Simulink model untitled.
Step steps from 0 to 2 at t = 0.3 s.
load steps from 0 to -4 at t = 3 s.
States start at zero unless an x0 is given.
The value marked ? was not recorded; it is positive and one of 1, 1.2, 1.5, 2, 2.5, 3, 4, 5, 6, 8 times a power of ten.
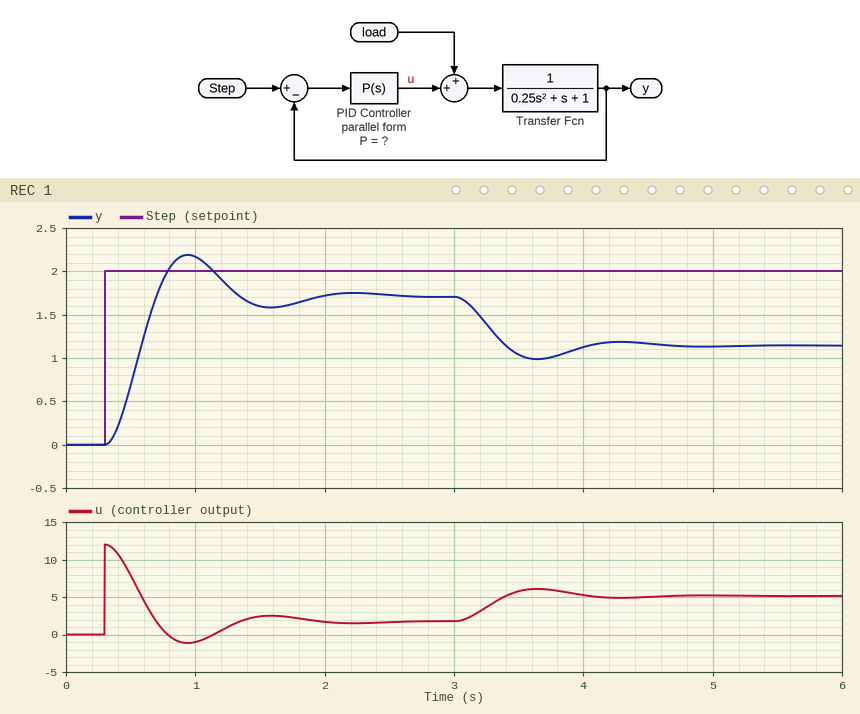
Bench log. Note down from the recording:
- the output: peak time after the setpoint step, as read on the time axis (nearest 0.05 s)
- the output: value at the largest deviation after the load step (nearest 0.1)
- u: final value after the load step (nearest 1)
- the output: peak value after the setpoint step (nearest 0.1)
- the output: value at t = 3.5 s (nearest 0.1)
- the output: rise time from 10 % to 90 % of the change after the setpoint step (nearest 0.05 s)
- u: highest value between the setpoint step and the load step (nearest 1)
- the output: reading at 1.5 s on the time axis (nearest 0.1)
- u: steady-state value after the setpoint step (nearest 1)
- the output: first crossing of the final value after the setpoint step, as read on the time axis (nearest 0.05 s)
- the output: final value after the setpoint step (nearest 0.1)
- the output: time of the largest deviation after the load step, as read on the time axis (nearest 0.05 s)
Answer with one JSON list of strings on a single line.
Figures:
["0.95 s", "1.0", "5", "2.2", "1.0", "0.25 s", "12", "1.6", "2", "0.70 s", "1.7", "3.65 s"]
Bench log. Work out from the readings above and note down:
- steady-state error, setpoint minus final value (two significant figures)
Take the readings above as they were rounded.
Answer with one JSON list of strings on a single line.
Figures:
["0.30"]
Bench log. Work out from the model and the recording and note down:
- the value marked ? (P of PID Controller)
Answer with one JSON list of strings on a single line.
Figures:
["6"]
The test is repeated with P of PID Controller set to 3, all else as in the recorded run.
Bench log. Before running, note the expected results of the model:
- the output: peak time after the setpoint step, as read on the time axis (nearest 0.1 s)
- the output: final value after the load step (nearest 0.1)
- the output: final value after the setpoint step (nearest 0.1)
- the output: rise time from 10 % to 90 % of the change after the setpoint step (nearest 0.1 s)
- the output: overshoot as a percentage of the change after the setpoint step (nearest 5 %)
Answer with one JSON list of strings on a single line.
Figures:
["1.2 s", "0.5", "1.5", "0.4 s", "15 %"]
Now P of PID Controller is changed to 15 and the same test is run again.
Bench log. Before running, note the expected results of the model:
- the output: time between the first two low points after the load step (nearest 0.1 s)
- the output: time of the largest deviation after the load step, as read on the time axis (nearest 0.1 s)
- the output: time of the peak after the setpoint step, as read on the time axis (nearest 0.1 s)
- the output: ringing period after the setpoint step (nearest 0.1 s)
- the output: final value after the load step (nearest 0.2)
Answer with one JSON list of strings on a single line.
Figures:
["0.8 s", "3.4 s", "0.7 s", "0.8 s", "1.6"]
